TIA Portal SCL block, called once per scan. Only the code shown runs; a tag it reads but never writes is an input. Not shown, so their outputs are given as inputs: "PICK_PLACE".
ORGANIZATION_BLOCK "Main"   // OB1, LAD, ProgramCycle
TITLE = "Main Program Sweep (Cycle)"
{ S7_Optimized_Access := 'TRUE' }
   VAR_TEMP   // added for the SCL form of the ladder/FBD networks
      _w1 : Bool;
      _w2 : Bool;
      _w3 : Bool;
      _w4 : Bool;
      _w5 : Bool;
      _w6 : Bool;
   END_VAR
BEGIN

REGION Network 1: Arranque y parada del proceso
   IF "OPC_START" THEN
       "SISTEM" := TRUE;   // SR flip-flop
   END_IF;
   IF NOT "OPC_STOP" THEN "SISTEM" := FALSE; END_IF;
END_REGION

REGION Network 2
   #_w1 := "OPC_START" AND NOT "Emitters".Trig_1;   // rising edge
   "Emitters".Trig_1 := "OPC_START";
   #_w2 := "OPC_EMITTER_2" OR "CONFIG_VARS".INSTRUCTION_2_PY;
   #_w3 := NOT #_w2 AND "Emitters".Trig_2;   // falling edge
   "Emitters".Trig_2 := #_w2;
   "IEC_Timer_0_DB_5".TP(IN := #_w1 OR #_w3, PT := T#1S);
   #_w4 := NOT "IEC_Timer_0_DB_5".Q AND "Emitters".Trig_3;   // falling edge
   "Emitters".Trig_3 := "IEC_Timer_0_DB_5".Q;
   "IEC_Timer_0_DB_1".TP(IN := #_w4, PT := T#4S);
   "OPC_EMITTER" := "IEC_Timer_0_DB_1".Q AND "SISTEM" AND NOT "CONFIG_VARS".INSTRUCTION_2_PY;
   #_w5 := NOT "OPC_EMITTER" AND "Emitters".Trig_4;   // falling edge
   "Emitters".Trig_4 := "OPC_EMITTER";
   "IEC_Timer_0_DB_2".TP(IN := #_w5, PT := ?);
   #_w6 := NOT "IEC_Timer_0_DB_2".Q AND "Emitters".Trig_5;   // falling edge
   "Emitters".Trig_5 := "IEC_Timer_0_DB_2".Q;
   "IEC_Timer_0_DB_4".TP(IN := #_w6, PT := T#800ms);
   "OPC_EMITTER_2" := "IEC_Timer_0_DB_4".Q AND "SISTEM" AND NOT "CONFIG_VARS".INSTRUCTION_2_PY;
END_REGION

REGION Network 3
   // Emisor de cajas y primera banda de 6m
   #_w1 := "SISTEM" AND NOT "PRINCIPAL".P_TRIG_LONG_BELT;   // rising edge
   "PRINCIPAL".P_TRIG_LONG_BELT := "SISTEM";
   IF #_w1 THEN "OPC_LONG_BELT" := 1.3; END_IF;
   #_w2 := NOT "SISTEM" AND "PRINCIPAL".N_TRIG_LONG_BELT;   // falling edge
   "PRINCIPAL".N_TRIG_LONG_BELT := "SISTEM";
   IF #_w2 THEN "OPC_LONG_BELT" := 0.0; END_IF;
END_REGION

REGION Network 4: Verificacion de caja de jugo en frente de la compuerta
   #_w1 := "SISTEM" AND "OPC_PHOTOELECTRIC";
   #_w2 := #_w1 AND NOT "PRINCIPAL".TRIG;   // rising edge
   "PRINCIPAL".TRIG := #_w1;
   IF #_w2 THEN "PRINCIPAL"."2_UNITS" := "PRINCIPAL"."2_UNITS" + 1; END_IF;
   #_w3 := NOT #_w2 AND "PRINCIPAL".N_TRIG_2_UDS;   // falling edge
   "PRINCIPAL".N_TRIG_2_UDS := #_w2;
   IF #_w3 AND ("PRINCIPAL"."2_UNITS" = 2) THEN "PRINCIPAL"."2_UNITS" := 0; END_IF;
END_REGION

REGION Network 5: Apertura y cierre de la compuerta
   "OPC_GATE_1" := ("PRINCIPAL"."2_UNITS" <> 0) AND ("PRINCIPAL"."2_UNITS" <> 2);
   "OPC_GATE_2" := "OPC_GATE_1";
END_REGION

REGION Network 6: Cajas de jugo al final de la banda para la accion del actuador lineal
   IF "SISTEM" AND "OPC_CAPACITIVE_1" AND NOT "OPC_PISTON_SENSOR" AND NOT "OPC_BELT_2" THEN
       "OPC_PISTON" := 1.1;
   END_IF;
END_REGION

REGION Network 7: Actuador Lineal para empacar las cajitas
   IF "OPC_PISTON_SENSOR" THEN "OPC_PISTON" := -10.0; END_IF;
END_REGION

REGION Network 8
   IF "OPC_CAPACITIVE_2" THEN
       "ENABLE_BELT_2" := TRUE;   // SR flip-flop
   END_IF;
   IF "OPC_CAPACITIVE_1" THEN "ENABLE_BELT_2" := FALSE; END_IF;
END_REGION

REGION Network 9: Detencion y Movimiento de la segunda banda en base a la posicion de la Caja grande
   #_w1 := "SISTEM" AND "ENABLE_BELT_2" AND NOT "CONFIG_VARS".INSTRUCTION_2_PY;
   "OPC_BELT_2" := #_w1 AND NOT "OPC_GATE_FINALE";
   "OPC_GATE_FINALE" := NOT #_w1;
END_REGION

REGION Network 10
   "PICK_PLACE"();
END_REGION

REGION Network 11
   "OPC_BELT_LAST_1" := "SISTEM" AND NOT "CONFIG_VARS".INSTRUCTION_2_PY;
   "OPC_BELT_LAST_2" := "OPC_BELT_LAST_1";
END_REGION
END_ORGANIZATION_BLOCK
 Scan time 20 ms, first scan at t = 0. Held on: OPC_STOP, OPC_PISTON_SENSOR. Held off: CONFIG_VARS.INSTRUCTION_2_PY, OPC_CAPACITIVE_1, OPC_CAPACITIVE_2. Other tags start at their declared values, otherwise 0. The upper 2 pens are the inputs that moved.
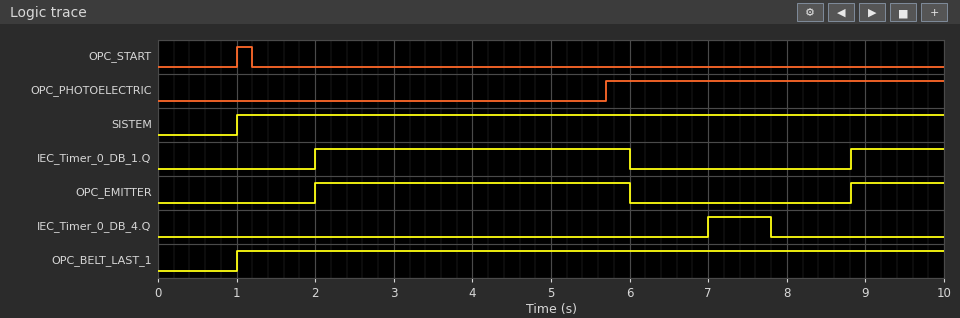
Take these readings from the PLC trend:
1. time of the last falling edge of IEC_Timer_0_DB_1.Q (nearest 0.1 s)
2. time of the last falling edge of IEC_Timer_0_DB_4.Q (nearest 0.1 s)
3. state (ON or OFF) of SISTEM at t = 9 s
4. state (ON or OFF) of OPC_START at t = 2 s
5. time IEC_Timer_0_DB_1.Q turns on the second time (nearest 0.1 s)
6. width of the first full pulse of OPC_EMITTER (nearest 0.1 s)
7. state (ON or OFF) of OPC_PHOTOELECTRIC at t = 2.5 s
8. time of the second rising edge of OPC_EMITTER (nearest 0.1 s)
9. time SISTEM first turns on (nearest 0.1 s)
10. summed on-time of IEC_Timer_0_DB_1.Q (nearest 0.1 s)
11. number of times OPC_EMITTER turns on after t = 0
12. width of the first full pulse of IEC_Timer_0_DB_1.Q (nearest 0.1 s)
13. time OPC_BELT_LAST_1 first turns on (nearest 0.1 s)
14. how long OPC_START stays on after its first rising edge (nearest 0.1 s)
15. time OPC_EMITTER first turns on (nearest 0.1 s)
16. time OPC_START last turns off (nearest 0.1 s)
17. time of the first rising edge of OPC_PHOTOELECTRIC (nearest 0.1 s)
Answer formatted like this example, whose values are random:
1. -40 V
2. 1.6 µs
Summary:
1. 6.0 s
2. 7.8 s
3. ON
4. OFF
5. 8.8 s
6. 4.0 s
7. OFF
8. 8.8 s
9. 1.0 s
10. 5.2 s
11. 2
12. 4.0 s
13. 1.0 s
14. 0.2 s
15. 2.0 s
16. 1.2 s
17. 5.7 s
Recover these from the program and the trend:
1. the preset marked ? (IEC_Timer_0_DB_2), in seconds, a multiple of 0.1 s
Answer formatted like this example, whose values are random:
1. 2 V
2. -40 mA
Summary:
1. 1.0 s
